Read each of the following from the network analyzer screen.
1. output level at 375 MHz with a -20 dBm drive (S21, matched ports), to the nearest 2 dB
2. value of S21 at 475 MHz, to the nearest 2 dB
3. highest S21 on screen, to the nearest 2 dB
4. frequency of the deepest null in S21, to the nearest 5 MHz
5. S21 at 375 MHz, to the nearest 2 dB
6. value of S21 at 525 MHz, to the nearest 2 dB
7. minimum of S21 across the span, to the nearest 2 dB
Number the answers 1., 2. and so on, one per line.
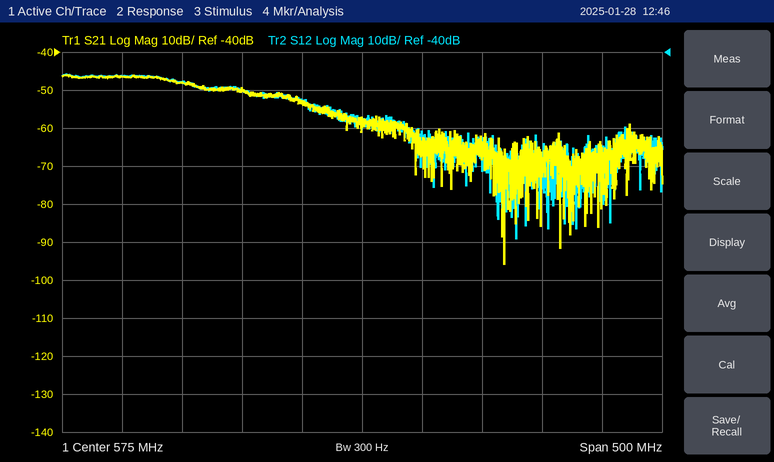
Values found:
1. -66 dBm
2. -50 dB
3. -46 dB
4. 695 MHz
5. -46 dB
6. -54 dB
7. -96 dB
